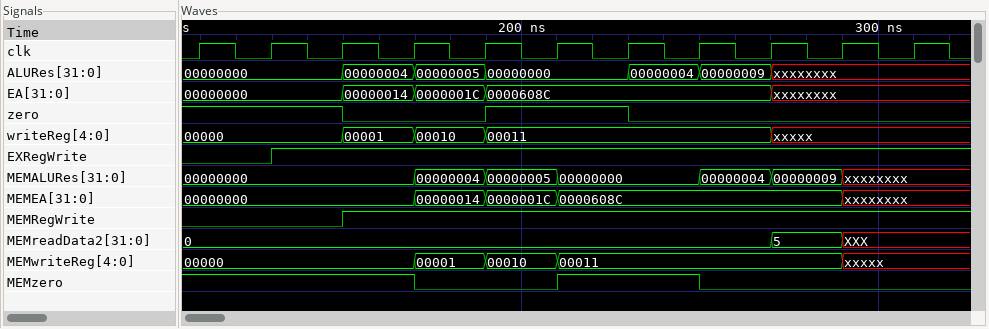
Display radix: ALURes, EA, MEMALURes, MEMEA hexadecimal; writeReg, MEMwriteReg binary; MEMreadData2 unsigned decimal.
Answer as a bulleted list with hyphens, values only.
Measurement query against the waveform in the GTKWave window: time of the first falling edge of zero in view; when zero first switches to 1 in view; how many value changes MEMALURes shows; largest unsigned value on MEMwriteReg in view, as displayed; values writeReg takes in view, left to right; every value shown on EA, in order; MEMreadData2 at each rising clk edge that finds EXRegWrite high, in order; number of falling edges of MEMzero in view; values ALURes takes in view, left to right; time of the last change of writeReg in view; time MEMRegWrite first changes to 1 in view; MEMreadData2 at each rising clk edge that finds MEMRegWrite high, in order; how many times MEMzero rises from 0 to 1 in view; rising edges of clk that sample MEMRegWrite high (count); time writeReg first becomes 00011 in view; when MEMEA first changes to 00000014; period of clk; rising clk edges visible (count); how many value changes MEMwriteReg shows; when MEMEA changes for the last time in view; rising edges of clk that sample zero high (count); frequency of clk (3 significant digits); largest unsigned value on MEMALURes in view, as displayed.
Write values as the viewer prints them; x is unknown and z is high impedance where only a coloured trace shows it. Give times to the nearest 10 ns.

- 150 ns
- 190 ns
- 6
- 00011
- 00000, 00001, 00010, 00011, xxxxx
- 00000000, 00000014, 0000001C, 0000608C, xxxxxxxx
- 0, 0, 0, 0, 0, 0, 0, 5, XXX
- 2
- 00000000, 00000004, 00000005, 00000000, 00000004, 00000009, xxxxxxxx
- 270 ns
- 150 ns
- 0, 0, 0, 0, 0, 0, 5, XXX
- 1
- 8
- 190 ns
- 170 ns
- 20 ns
- 11
- 4
- 290 ns
- 5
- 50.0 MHz
- 00000009
